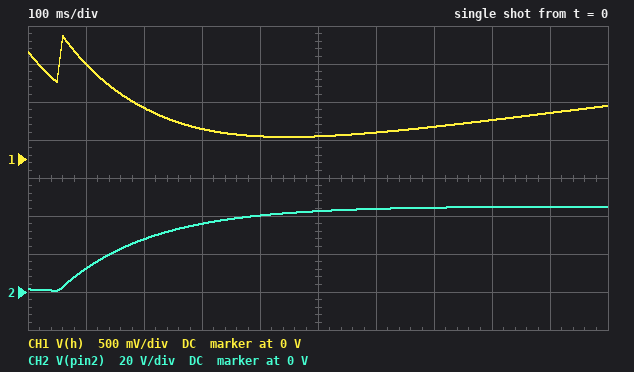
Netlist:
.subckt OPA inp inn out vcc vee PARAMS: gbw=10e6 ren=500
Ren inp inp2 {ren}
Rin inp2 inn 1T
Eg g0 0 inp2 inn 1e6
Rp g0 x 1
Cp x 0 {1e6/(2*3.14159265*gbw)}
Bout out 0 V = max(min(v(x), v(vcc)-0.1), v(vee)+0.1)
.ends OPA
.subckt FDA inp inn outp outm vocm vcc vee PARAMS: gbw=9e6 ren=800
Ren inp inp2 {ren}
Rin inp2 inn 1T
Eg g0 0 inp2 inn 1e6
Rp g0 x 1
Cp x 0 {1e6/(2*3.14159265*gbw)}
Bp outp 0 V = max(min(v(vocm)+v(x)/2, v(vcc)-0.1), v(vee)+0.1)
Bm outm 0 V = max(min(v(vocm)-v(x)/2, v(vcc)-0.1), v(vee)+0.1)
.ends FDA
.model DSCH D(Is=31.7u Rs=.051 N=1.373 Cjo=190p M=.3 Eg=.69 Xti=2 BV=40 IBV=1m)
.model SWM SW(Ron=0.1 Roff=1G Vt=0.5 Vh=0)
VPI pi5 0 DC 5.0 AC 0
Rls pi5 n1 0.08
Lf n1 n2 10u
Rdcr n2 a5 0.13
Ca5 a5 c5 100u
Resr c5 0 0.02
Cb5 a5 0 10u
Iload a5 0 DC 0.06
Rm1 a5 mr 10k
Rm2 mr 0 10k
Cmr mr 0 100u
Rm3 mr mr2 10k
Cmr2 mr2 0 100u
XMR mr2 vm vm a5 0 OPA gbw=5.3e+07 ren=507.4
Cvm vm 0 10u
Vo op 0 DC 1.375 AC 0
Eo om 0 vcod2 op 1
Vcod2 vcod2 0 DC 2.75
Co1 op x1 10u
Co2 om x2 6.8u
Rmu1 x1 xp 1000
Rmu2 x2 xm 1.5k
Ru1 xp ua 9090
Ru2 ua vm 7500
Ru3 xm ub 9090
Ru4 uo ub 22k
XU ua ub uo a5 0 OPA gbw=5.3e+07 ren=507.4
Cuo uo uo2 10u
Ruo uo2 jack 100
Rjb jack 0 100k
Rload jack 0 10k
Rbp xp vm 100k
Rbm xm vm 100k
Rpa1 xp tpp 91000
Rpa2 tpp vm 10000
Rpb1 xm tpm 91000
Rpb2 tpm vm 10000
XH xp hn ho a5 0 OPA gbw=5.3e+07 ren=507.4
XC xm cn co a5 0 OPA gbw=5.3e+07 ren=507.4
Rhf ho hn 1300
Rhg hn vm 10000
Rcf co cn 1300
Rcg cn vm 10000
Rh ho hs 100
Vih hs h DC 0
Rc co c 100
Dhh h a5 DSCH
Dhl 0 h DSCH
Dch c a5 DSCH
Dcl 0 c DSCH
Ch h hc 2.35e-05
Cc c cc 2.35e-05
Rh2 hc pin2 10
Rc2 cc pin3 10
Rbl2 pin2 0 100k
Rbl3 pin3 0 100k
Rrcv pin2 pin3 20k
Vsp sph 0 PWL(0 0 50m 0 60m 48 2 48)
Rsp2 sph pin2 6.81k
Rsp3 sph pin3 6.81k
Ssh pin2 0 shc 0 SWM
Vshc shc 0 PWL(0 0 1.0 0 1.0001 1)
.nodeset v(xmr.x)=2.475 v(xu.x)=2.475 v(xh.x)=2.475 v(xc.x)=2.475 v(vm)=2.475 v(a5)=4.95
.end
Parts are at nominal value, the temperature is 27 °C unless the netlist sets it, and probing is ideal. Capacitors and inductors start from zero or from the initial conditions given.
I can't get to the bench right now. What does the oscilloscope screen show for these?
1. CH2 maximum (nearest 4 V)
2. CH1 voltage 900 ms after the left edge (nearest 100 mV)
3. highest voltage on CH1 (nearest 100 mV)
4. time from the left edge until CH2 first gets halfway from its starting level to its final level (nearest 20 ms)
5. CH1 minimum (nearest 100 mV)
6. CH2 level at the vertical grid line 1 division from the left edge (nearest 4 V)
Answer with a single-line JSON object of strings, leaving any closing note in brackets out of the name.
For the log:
{"CH2 maximum": "44 V", "CH1 voltage 900 ms after the left edge": "600 mV", "highest voltage on CH1": "1.6 V", "time from the left edge until CH2 first gets halfway from its starting level to its final level": "160 ms", "CH1 minimum": "300 mV", "CH2 level at the vertical grid line 1 division from the left edge": "12 V"}
